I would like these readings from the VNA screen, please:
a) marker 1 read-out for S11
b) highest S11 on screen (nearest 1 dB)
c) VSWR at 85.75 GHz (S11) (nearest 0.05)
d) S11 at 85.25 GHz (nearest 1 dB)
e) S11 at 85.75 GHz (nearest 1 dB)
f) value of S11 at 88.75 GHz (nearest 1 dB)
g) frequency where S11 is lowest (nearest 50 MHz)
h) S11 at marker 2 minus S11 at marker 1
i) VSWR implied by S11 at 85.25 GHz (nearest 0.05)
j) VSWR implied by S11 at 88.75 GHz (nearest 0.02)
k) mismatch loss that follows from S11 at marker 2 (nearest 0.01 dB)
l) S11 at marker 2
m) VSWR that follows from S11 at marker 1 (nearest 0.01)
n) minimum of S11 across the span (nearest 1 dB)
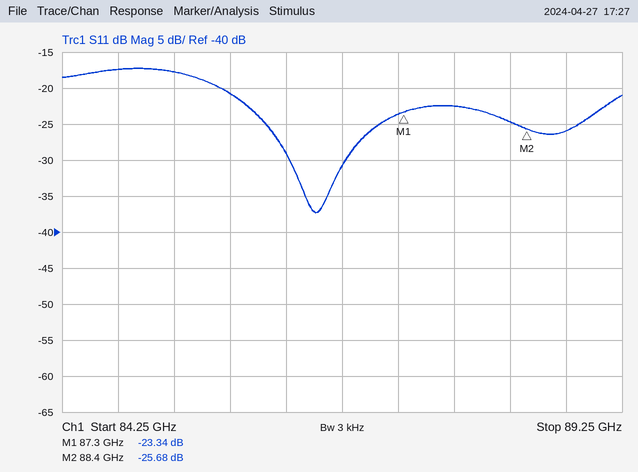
-23.34 dB
-17 dB
1.20
-18 dB
-21 dB
-26 dB
86.50 GHz
-2.34 dB
1.30
1.10
0.01 dB
-25.68 dB
1.15
-37 dB
